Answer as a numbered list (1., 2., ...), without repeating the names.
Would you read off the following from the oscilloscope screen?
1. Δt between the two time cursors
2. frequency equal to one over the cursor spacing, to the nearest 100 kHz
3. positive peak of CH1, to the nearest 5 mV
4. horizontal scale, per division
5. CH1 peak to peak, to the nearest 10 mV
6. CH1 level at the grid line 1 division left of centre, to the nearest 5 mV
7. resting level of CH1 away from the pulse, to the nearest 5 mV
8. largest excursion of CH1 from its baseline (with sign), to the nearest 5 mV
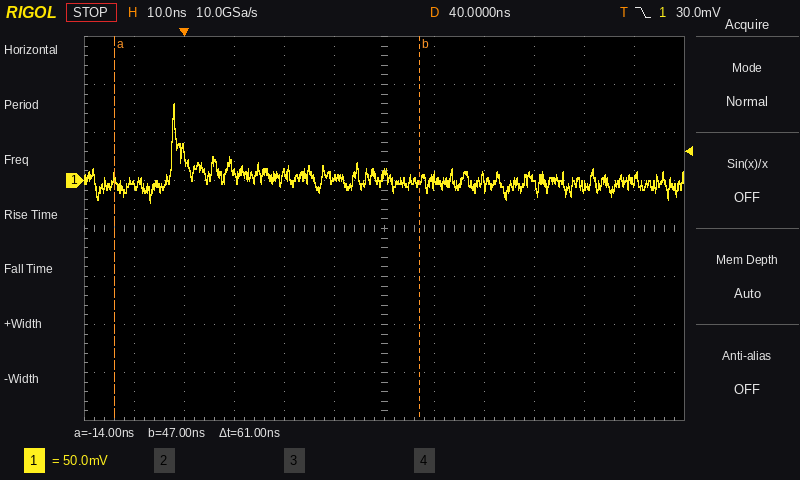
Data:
1. 61 ns
2. 16.4 MHz
3. 80 mV
4. 10 ns
5. 100 mV
6. 0 mV
7. 0 mV
8. +80 mV
